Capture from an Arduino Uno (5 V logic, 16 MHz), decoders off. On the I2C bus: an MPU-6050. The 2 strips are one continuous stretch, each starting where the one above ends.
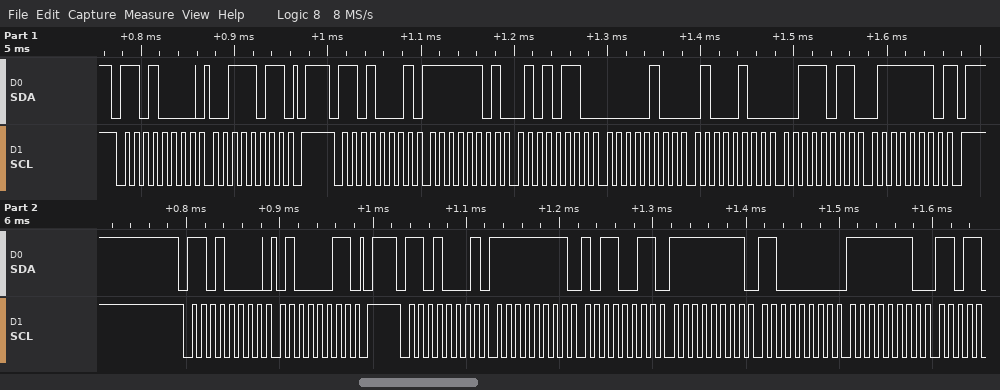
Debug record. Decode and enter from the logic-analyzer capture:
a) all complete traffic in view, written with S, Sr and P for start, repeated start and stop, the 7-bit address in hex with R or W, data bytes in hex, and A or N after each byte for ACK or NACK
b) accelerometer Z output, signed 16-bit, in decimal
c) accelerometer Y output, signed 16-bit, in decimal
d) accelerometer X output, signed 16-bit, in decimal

S 68W A 3B A P S 68R A FD A 56 A 04 A 44 A 3B A 7E N P S 68W A 43 A P S 68R A FF A B3 A FF A C0 A FE A
15230
1092
-682
